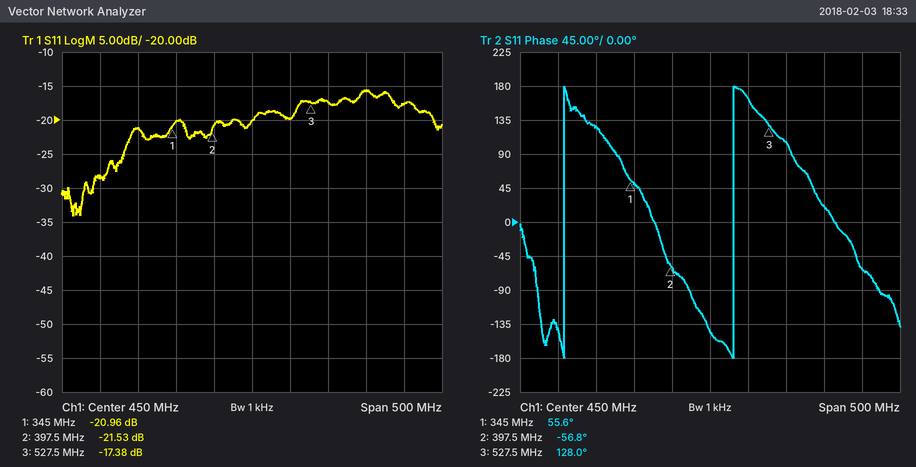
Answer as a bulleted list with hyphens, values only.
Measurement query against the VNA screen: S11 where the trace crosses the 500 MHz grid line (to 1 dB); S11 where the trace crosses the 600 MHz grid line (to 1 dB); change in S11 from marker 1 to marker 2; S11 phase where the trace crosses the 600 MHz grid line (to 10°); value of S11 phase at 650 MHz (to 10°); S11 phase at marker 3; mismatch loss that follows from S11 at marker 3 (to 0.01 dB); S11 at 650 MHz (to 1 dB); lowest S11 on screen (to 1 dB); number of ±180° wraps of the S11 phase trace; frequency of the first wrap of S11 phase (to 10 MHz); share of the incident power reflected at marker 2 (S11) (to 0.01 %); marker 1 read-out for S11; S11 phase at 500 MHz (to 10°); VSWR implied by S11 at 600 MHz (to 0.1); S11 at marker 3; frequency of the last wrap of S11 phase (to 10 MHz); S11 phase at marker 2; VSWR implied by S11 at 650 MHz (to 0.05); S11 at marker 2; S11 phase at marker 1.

- -20 dB
- -16 dB
- -0.57 dB
- 20°
- -60°
- 128.0°
- 0.08 dB
- -18 dB
- -34 dB
- 2
- 260 MHz
- 0.70 %
- -20.96 dB
- 160°
- 1.4
- -17.38 dB
- 480 MHz
- -56.8°
- 1.30
- -21.53 dB
- 55.6°
